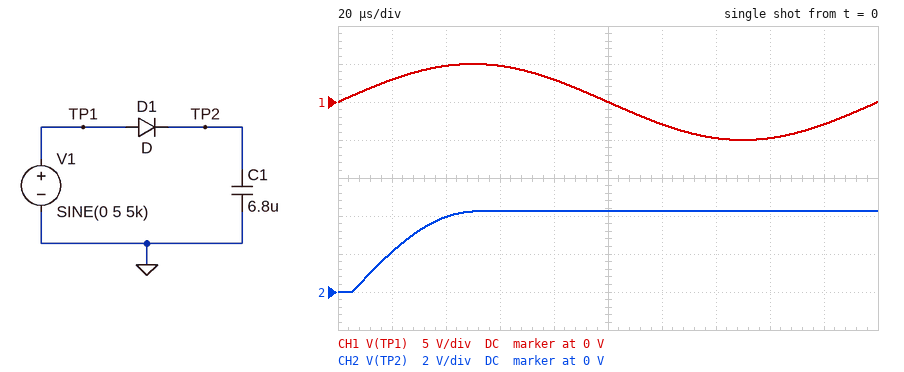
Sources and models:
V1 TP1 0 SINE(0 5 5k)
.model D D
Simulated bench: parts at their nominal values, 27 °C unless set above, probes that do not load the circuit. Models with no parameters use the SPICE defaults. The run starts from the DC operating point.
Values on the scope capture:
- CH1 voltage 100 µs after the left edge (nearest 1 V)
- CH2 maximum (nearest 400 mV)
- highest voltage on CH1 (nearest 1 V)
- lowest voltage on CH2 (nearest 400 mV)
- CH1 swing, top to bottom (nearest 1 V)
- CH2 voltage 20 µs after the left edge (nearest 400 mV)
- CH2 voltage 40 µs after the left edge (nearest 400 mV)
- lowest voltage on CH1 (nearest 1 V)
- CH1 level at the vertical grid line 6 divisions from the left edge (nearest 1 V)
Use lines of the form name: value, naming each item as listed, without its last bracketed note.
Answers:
CH1 voltage 100 µs after the left edge: 0 V
CH2 maximum: 4.4 V
highest voltage on CH1: 5 V
lowest voltage on CH2: 0 V
CH1 swing, top to bottom: 10 V
CH2 voltage 20 µs after the left edge: 2.0 V
CH2 voltage 40 µs after the left edge: 4.0 V
lowest voltage on CH1: -5 V
CH1 level at the vertical grid line 6 divisions from the left edge: -3 V
